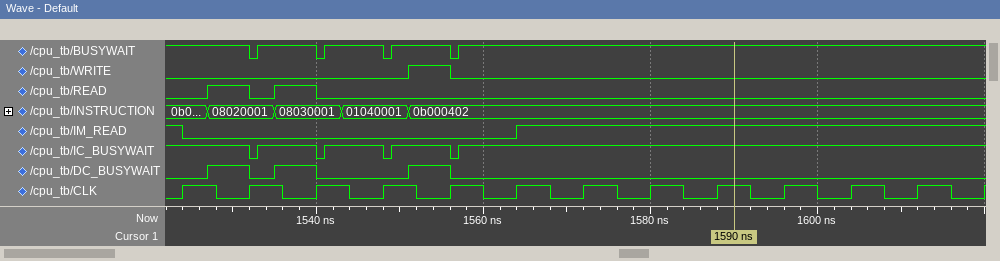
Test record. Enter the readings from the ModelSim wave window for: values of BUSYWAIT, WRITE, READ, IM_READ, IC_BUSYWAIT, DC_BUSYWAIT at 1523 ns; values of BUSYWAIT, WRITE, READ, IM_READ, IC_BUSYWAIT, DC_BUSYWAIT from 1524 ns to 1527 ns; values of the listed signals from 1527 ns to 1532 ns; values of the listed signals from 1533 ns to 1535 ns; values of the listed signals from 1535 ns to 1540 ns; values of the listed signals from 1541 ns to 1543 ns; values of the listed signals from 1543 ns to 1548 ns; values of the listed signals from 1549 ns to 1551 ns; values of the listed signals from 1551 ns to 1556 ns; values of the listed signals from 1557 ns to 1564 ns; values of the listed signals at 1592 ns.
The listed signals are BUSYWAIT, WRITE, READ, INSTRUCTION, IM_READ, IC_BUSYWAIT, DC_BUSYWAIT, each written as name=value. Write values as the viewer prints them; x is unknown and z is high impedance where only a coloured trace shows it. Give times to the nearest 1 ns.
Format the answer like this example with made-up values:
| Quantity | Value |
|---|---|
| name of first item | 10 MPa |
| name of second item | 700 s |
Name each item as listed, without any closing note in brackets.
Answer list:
| Quantity | Value |
|---|---|
| values of BUSYWAIT, WRITE, READ, IM_READ, IC_BUSYWAIT, DC_BUSYWAIT at 1523 ns | BUSYWAIT=1, WRITE=0, READ=0, IM_READ=1, IC_BUSYWAIT=1, DC_BUSYWAIT=0 |
| values of BUSYWAIT, WRITE, READ, IM_READ, IC_BUSYWAIT, DC_BUSYWAIT from 1524 ns to 1527 ns | BUSYWAIT=1, WRITE=0, READ=0, IM_READ=0, IC_BUSYWAIT=1, DC_BUSYWAIT=0 |
| values of the listed signals from 1527 ns to 1532 ns | BUSYWAIT=1, WRITE=0, READ=1, INSTRUCTION=08020001, IM_READ=0, IC_BUSYWAIT=1, DC_BUSYWAIT=1 |
| values of the listed signals from 1533 ns to 1535 ns | BUSYWAIT=1, WRITE=0, READ=0, INSTRUCTION=08020001, IM_READ=0, IC_BUSYWAIT=1, DC_BUSYWAIT=0 |
| values of the listed signals from 1535 ns to 1540 ns | BUSYWAIT=1, WRITE=0, READ=1, INSTRUCTION=08030001, IM_READ=0, IC_BUSYWAIT=1, DC_BUSYWAIT=1 |
| values of the listed signals from 1541 ns to 1543 ns | BUSYWAIT=1, WRITE=0, READ=0, INSTRUCTION=08030001, IM_READ=0, IC_BUSYWAIT=1, DC_BUSYWAIT=0 |
| values of the listed signals from 1543 ns to 1548 ns | BUSYWAIT=1, WRITE=0, READ=0, INSTRUCTION=01040001, IM_READ=0, IC_BUSYWAIT=1, DC_BUSYWAIT=0 |
| values of the listed signals from 1549 ns to 1551 ns | BUSYWAIT=1, WRITE=0, READ=0, INSTRUCTION=01040001, IM_READ=0, IC_BUSYWAIT=1, DC_BUSYWAIT=0 |
| values of the listed signals from 1551 ns to 1556 ns | BUSYWAIT=1, WRITE=1, READ=0, INSTRUCTION=0b000402, IM_READ=0, IC_BUSYWAIT=1, DC_BUSYWAIT=1 |
| values of the listed signals from 1557 ns to 1564 ns | BUSYWAIT=1, WRITE=0, READ=0, INSTRUCTION=0b000402, IM_READ=0, IC_BUSYWAIT=1, DC_BUSYWAIT=0 |
| values of the listed signals at 1592 ns | BUSYWAIT=1, WRITE=0, READ=0, INSTRUCTION=0b000402, IM_READ=1, IC_BUSYWAIT=1, DC_BUSYWAIT=0 |
